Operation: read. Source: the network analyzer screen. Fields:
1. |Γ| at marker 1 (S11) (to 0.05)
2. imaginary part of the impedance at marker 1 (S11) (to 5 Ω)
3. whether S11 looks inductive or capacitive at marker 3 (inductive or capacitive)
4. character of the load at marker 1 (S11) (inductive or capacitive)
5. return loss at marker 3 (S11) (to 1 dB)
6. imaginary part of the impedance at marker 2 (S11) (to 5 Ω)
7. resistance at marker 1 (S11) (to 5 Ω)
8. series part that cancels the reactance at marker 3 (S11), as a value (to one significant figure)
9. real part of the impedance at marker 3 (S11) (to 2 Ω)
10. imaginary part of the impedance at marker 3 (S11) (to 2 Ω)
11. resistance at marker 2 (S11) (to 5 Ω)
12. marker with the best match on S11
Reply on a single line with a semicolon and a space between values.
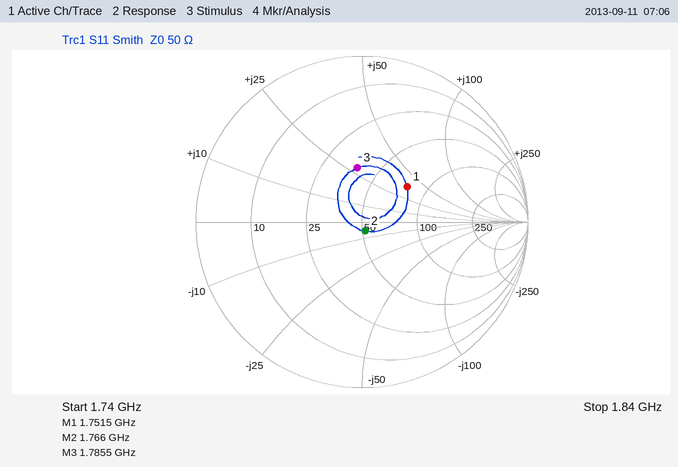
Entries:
0.35; +35 Ω; inductive; inductive; 10 dB; -5 Ω; 75 Ω; 3 pF; 38 Ω; +28 Ω; 50 Ω; marker 2
